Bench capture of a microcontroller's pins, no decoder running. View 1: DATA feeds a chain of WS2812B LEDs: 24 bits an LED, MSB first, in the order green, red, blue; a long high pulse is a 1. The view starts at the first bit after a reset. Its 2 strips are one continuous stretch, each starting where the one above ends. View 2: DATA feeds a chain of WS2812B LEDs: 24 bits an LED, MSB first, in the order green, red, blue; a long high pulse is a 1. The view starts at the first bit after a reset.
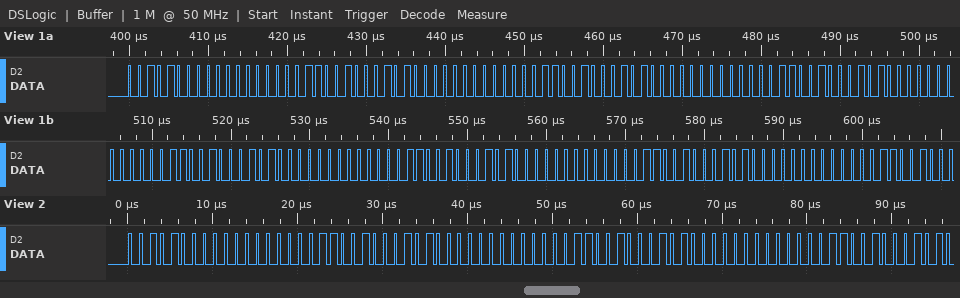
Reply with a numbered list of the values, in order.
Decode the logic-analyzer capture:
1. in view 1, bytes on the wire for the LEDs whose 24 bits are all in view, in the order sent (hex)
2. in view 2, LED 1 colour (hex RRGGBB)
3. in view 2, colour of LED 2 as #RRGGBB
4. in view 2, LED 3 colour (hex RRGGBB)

1. 28 00 32 28 00 32 28 00 32 28 00 32 28 00 32 28 00 32 28 00 32
2. #002832
3. #002832
4. #002832
